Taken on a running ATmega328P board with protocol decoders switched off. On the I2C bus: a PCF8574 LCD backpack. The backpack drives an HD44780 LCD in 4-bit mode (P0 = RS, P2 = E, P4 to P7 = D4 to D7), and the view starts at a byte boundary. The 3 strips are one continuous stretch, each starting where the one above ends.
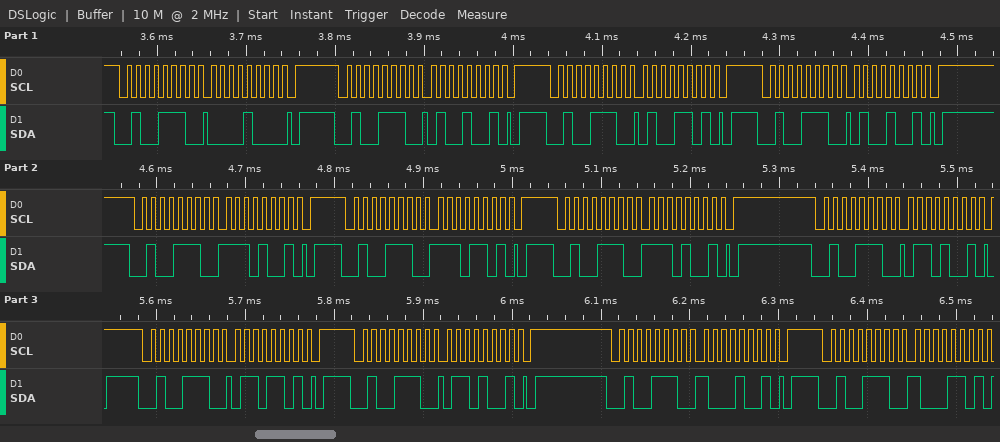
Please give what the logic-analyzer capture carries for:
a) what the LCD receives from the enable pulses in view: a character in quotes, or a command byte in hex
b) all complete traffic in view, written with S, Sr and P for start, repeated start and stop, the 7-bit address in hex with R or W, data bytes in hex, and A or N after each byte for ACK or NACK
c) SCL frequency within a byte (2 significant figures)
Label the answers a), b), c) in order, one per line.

a) 'N'
b) S 27W A 08 A P S 27W A 49 A P S 27W A 4D A P S 27W A 49 A P S 27W A E9 A P S 27W A ED A P S 27W A E9 A P S 27W A 69 A P S 27W A 6D A P S 27W A 69 A P S 27W A 89 A P S 27W A 8D A
c) 100 kHz
